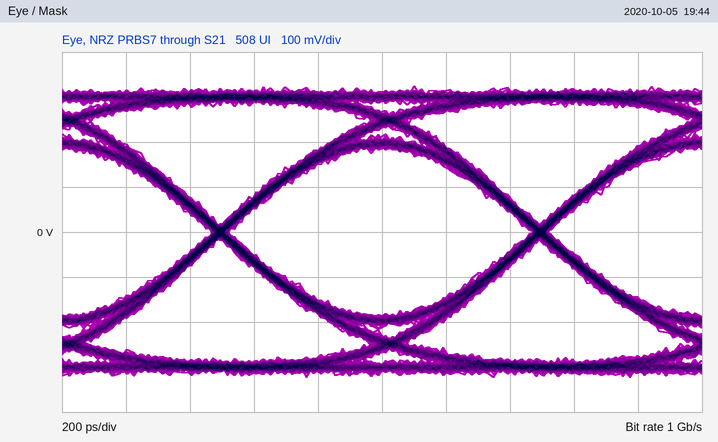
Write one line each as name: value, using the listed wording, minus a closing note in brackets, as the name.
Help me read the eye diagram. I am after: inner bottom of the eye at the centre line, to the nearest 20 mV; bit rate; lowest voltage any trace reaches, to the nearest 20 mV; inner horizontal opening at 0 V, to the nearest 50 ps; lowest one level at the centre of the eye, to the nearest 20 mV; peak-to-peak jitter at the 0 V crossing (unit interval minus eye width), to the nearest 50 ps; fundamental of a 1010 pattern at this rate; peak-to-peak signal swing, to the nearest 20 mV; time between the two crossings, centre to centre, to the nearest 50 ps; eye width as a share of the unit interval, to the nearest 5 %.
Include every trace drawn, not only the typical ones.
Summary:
inner bottom of the eye at the centre line, to the nearest 20 mV: -180 mV
bit rate: 1 Gb/s
lowest voltage any trace reaches, to the nearest 20 mV: -320 mV
inner horizontal opening at 0 V, to the nearest 50 ps: 950 ps
lowest one level at the centre of the eye, to the nearest 20 mV: 180 mV
peak-to-peak jitter at the 0 V crossing (unit interval minus eye width), to the nearest 50 ps: 50 ps
fundamental of a 1010 pattern at this rate: 500 MHz
peak-to-peak signal swing, to the nearest 20 mV: 640 mV
time between the two crossings, centre to centre, to the nearest 50 ps: 1.00 ns
eye width as a share of the unit interval, to the nearest 5 %: 95 %
